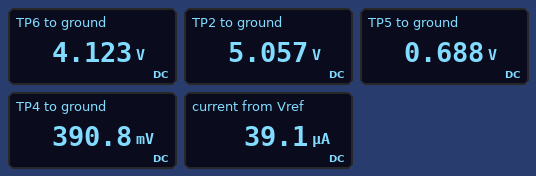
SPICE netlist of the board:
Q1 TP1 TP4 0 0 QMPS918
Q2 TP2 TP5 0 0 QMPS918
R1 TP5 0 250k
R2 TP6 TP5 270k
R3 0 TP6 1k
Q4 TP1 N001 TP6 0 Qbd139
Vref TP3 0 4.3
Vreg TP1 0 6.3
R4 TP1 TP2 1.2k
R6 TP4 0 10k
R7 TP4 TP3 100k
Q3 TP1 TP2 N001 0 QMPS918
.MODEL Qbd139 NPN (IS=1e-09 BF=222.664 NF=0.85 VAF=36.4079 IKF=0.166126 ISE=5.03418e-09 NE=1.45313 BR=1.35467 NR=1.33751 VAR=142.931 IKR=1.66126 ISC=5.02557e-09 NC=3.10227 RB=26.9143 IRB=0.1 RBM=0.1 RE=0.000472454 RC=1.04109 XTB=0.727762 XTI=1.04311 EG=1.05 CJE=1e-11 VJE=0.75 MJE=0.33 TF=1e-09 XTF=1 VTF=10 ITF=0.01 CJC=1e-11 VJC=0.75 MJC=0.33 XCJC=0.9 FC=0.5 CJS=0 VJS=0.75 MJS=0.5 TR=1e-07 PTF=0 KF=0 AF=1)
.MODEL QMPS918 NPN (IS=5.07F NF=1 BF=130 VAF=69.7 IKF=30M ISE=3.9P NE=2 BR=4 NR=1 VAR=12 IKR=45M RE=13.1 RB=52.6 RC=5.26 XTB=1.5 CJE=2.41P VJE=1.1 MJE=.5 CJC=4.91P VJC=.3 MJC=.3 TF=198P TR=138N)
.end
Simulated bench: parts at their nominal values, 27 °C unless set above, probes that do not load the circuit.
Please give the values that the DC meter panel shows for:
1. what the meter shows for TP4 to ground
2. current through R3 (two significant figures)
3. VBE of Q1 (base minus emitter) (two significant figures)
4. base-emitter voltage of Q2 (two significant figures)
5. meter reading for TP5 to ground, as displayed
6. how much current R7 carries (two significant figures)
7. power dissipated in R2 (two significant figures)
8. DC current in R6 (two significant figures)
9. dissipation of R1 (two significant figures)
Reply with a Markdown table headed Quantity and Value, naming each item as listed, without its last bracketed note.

| Quantity | Value |
|---|---|
| what the meter shows for TP4 to ground | 390.8 mV |
| current through R3 | 4.1 mA |
| VBE of Q1 (base minus emitter) | 390 mV |
| base-emitter voltage of Q2 | 690 mV |
| meter reading for TP5 to ground, as displayed | 0.688 V |
| how much current R7 carries | 39 µA |
| power dissipated in R2 | 44 µW |
| DC current in R6 | 39 µA |
| dissipation of R1 | 1.9 µW |
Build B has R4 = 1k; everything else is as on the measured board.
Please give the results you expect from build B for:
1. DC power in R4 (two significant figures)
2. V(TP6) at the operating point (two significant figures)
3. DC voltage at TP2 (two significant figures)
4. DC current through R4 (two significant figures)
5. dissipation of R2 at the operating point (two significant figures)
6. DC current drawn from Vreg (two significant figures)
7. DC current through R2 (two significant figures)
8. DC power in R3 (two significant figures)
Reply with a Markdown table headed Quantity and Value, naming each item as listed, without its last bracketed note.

| Quantity | Value |
|---|---|
| DC power in R4 | 1.2 mW |
| V(TP6) at the operating point | 4.3 V |
| DC voltage at TP2 | 5.2 V |
| DC current through R4 | 1.1 mA |
| dissipation of R2 at the operating point | 47 µW |
| DC current drawn from Vreg | 5.4 mA |
| DC current through R2 | 13 µA |
| DC power in R3 | 18 mW |
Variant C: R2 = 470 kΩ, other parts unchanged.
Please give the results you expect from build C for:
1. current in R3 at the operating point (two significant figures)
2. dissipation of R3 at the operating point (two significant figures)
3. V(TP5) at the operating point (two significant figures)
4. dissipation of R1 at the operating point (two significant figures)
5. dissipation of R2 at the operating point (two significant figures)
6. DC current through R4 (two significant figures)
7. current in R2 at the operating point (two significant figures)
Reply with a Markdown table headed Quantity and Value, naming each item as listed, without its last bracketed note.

| Quantity | Value |
|---|---|
| current in R3 at the operating point | 4.7 mA |
| dissipation of R3 at the operating point | 22 mW |
| V(TP5) at the operating point | 670 mV |
| dissipation of R1 at the operating point | 1.8 µW |
| dissipation of R2 at the operating point | 34 µW |
| DC current through R4 | 580 µA |
| current in R2 at the operating point | 8.5 µA |
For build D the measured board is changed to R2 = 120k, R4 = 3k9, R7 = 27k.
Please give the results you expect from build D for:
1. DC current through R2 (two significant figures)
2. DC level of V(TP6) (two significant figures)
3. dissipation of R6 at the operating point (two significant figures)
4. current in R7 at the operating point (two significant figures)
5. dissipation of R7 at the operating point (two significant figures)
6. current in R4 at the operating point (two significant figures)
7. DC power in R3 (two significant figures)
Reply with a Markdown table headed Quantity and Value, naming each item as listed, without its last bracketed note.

| Quantity | Value |
|---|---|
| DC current through R2 | 11 µA |
| DC level of V(TP6) | 2.0 V |
| dissipation of R6 at the operating point | 63 µW |
| current in R7 at the operating point | 130 µA |
| dissipation of R7 at the operating point | 460 µW |
| current in R4 at the operating point | 860 µA |
| DC power in R3 | 4.2 mW |
